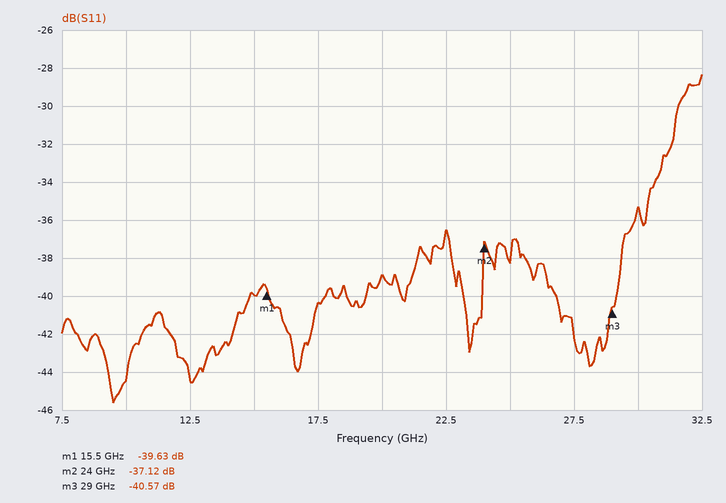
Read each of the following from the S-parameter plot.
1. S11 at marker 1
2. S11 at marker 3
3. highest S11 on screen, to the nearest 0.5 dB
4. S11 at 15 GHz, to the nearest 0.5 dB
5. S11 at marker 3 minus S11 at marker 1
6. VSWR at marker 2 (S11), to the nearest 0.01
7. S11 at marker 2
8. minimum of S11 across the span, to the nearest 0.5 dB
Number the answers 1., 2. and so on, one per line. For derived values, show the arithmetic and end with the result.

1. -39.63 dB
2. -40.57 dB
3. -28.5 dB
4. -40.0 dB
5. -40.57 − (-39.63) = -0.94 dB
6. (1 + 0.0139)/(1 − 0.0139) ≈ 1.03
7. -37.12 dB
8. -45.5 dB
